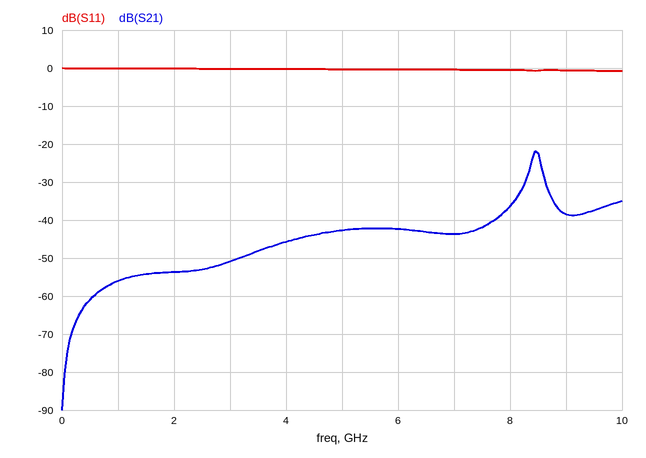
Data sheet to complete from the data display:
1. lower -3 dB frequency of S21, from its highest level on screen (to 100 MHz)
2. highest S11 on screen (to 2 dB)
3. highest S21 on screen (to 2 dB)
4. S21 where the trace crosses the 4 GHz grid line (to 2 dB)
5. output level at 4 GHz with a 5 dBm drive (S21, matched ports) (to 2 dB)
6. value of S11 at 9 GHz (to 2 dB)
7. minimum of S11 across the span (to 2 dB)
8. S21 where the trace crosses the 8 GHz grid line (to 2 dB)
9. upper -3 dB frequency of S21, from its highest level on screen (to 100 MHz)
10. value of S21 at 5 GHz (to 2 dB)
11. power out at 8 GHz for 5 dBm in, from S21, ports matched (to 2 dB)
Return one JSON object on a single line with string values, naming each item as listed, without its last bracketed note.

{"lower -3 dB frequency of S21, from its highest level on screen": "8.4 GHz", "highest S11 on screen": "0 dB", "highest S21 on screen": "-22 dB", "S21 where the trace crosses the 4 GHz grid line": "-46 dB", "output level at 4 GHz with a 5 dBm drive (S21, matched ports)": "-40 dBm", "value of S11 at 9 GHz": "0 dB", "minimum of S11 across the span": "0 dB", "S21 where the trace crosses the 8 GHz grid line": "-36 dB", "upper -3 dB frequency of S21, from its highest level on screen": "8.5 GHz", "value of S21 at 5 GHz": "-42 dB", "power out at 8 GHz for 5 dBm in, from S21, ports matched": "-32 dBm"}
